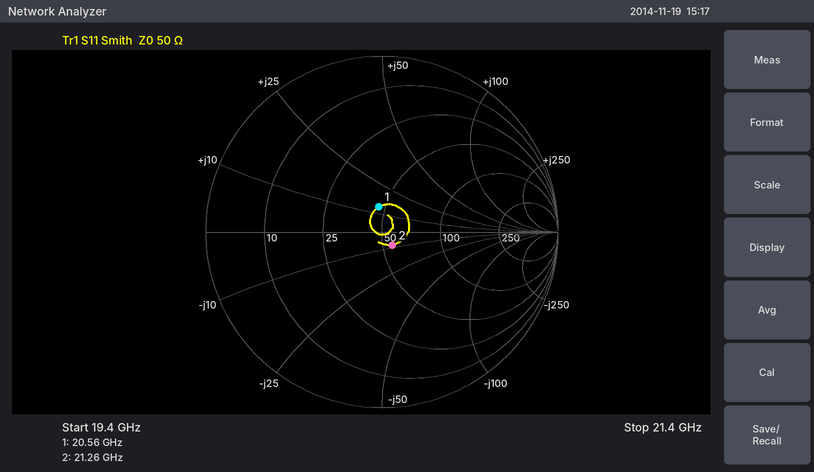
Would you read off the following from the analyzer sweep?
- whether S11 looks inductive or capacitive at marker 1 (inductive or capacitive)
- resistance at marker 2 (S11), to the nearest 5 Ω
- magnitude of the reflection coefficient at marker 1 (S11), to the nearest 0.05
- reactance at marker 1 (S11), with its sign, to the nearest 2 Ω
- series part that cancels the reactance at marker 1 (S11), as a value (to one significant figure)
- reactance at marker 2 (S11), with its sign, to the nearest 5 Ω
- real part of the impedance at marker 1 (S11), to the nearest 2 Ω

inductive
55 Ω
0.15
+14 Ω
600 fF
-10 Ω
46 Ω
